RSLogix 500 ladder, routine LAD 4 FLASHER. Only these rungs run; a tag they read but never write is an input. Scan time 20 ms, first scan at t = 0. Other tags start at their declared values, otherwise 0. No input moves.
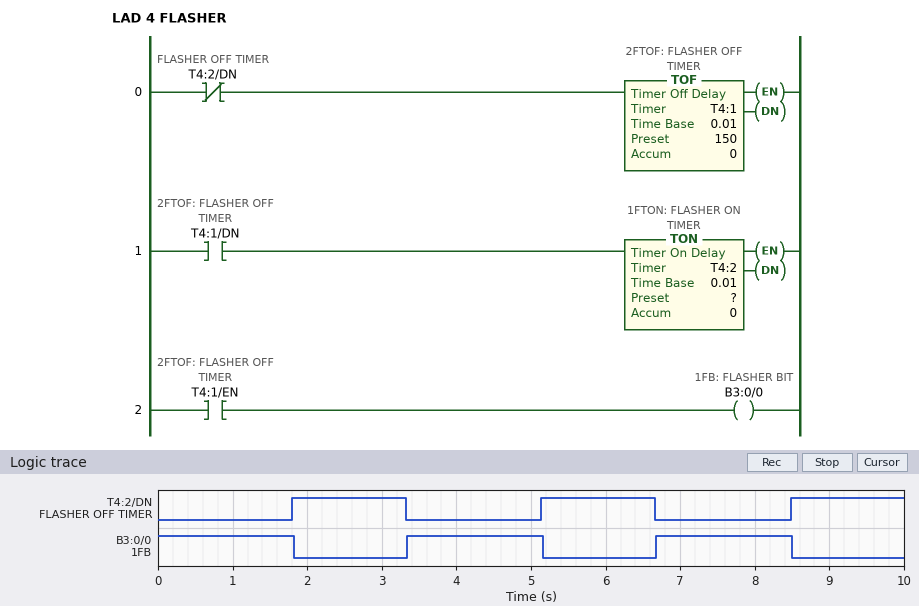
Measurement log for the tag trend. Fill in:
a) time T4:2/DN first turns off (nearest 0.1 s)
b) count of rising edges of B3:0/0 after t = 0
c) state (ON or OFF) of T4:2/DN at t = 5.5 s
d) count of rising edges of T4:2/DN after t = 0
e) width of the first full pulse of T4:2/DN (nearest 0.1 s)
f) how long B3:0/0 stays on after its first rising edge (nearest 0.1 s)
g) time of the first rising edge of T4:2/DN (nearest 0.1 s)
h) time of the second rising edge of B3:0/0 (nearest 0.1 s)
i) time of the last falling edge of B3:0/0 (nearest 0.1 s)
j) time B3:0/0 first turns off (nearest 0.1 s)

3.3 s
2
ON
3
1.5 s
1.8 s
1.8 s
6.7 s
8.5 s
1.8 s
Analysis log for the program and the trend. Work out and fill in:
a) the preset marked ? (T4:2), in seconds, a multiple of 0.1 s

1.8 s
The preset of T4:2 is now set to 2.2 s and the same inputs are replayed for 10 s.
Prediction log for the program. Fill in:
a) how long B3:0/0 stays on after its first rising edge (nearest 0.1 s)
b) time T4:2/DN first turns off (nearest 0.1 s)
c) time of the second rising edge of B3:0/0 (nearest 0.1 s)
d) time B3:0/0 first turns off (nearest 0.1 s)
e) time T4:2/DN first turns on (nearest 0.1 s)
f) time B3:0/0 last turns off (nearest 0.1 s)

2.2 s
3.7 s
7.5 s
2.2 s
2.2 s
9.7 s
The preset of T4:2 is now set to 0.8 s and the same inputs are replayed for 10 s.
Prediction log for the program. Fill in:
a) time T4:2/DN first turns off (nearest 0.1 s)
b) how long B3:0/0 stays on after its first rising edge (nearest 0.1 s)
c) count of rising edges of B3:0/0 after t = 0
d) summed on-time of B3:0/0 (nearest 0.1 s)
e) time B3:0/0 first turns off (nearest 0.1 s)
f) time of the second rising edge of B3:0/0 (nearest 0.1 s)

2.3 s
0.8 s
4
3.9 s
0.8 s
4.7 s
